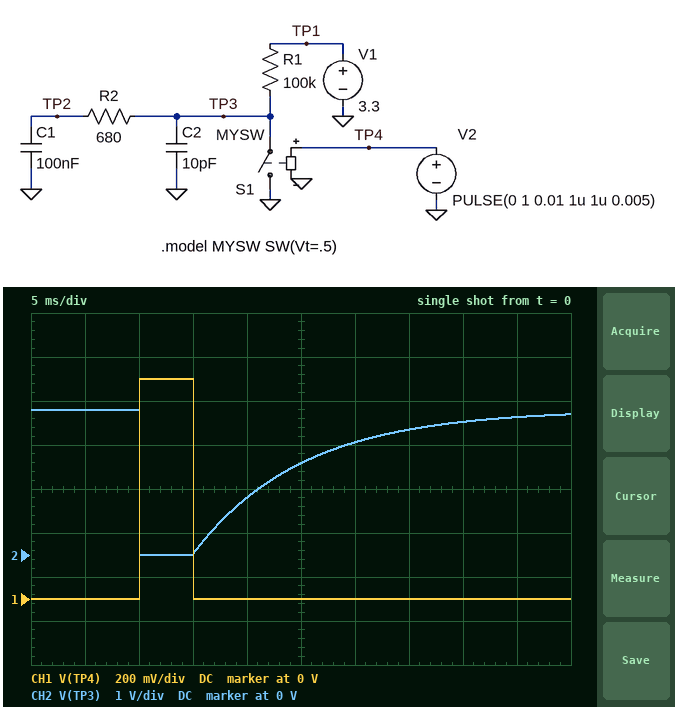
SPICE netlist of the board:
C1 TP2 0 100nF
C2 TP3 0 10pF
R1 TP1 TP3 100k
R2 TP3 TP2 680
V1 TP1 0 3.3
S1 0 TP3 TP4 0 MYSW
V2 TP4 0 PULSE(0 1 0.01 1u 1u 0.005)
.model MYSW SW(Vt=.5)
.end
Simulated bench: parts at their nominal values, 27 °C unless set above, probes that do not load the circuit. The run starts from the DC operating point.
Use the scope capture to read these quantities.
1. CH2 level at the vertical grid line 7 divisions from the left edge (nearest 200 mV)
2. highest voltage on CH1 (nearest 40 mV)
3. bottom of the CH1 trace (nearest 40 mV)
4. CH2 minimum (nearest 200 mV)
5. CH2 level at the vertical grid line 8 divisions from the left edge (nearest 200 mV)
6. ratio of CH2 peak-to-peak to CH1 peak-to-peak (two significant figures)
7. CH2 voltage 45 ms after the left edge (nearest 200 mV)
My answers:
2.8 V
1.00 V
0 V
0 V
3.0 V
3.3
3.2 V
